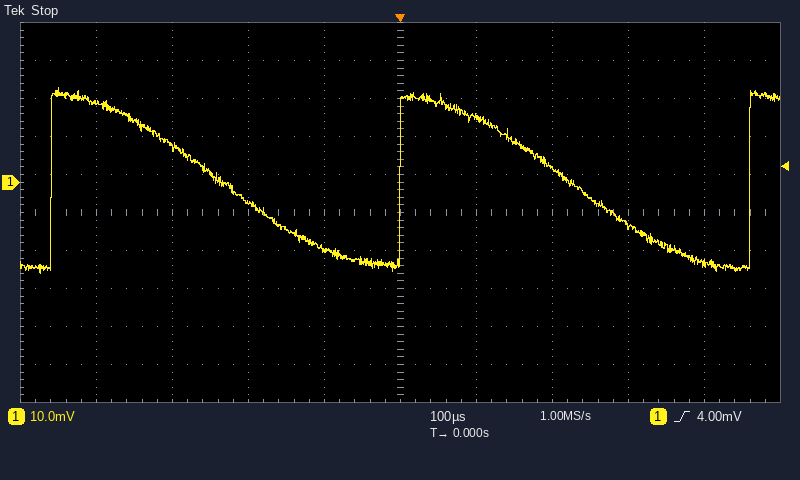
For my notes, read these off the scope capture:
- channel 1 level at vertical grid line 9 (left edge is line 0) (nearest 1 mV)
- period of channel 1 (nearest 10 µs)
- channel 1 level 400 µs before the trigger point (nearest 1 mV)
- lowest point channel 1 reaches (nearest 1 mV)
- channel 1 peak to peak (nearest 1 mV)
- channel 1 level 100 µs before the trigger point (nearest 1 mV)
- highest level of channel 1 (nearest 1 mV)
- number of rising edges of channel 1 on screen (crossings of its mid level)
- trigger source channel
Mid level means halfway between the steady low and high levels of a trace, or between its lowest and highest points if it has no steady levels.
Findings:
-21 mV
460 µs
21 mV
-24 mV
49 mV
-17 mV
25 mV
3
channel 1
